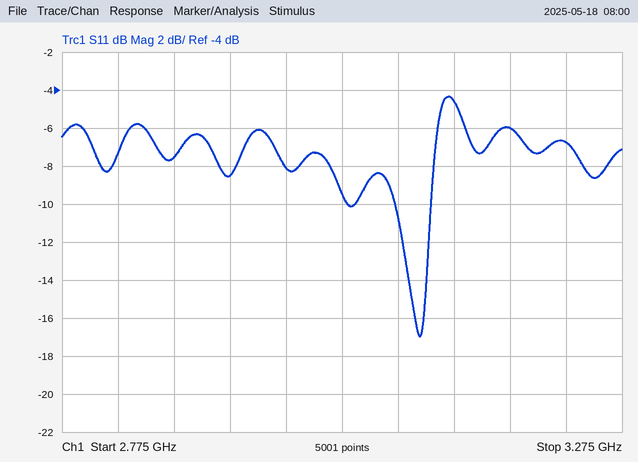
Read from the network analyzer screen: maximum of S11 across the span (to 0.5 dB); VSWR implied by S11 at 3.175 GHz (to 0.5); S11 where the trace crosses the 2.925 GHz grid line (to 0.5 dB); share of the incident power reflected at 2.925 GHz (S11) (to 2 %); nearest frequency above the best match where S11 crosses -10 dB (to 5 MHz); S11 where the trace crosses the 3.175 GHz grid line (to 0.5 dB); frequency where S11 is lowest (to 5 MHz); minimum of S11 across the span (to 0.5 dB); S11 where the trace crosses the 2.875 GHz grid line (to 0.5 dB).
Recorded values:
-4.5 dB
3.0
-8.5 dB
14 %
3.105 GHz
-6.0 dB
3.095 GHz
-17.0 dB
-7.5 dB
